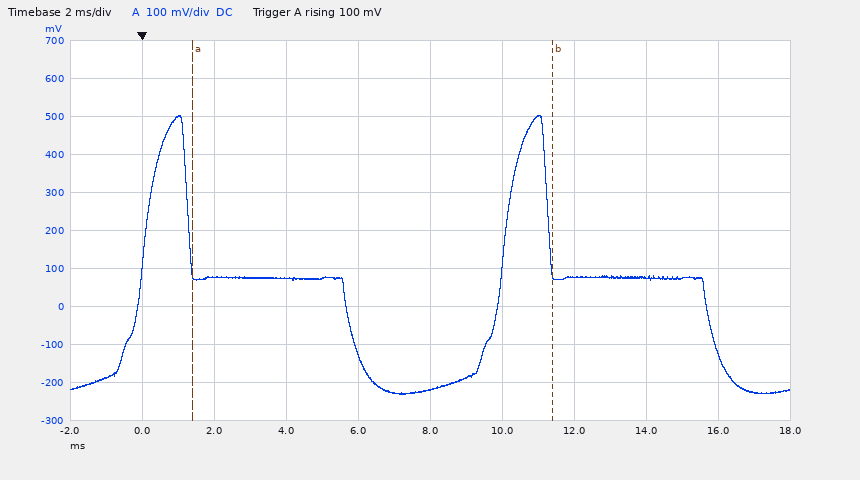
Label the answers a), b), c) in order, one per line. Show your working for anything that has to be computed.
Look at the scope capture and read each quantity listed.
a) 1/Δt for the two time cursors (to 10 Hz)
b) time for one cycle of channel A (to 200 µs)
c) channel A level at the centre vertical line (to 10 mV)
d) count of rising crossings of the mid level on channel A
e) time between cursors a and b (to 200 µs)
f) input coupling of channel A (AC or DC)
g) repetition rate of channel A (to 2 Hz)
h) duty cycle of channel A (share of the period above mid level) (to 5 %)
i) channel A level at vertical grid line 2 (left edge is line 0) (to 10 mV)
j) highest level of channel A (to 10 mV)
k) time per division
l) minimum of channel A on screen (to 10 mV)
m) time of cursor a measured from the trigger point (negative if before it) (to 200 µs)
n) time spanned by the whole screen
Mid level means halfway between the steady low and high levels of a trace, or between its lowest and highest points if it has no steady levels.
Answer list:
a) 1 / 10.0 ms ≈ 100 Hz
b) 10.0 ms
c) -220 mV
d) 2
e) 10.0 ms
f) DC
g) 1 / 10.0 ms ≈ 100 Hz
h) 15 %
i) 80 mV
j) 500 mV
k) 2 ms
l) -230 mV
m) +1.4 ms
n) 20 ms
